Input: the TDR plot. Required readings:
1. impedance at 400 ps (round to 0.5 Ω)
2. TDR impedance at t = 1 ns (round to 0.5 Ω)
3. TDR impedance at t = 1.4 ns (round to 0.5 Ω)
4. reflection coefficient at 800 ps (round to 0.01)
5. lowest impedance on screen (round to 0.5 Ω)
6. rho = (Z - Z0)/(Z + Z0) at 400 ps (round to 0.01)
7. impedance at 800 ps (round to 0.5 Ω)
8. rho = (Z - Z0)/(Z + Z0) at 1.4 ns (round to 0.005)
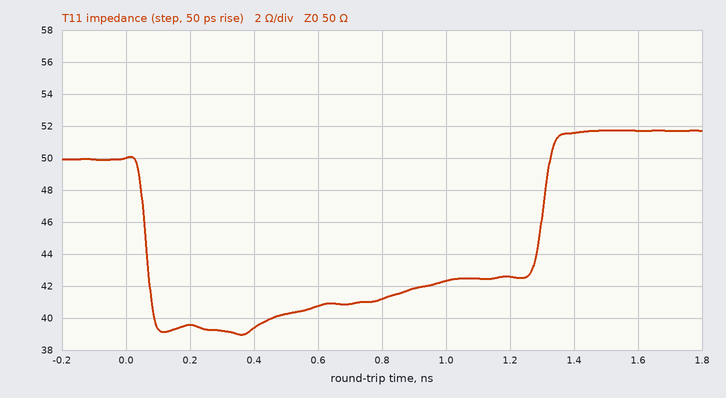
39.5 Ω
42.5 Ω
51.5 Ω
-0.10
39.0 Ω
-0.12
41.0 Ω
+0.015
